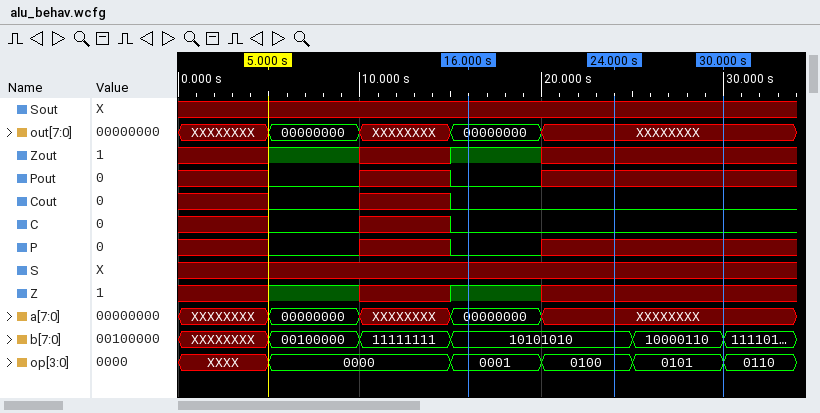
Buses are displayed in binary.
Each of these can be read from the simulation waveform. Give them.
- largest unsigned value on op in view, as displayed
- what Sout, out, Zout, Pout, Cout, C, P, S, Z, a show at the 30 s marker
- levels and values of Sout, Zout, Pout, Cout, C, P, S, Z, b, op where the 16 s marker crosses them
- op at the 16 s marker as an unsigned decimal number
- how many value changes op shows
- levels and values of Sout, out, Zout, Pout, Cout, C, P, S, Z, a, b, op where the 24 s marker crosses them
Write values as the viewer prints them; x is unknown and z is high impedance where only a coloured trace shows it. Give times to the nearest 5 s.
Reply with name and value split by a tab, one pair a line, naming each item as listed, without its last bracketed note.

largest unsigned value on op in view, as displayed	0110
what Sout, out, Zout, Pout, Cout, C, P, S, Z, a show at the 30 s marker	Sout=x, out=XXXXXXXX, Zout=x, Pout=x, Cout=0, C=0, P=x, S=x, Z=x, a=XXXXXXXX
levels and values of Sout, Zout, Pout, Cout, C, P, S, Z, b, op where the 16 s marker crosses them	Sout=x, Zout=1, Pout=0, Cout=0, C=0, P=0, S=x, Z=1, b=10101010, op=0001
op at the 16 s marker as an unsigned decimal number	1
how many value changes op shows	5
levels and values of Sout, out, Zout, Pout, Cout, C, P, S, Z, a, b, op where the 24 s marker crosses them	Sout=x, out=XXXXXXXX, Zout=x, Pout=x, Cout=0, C=0, P=x, S=x, Z=x, a=XXXXXXXX, b=10101010, op=0100
